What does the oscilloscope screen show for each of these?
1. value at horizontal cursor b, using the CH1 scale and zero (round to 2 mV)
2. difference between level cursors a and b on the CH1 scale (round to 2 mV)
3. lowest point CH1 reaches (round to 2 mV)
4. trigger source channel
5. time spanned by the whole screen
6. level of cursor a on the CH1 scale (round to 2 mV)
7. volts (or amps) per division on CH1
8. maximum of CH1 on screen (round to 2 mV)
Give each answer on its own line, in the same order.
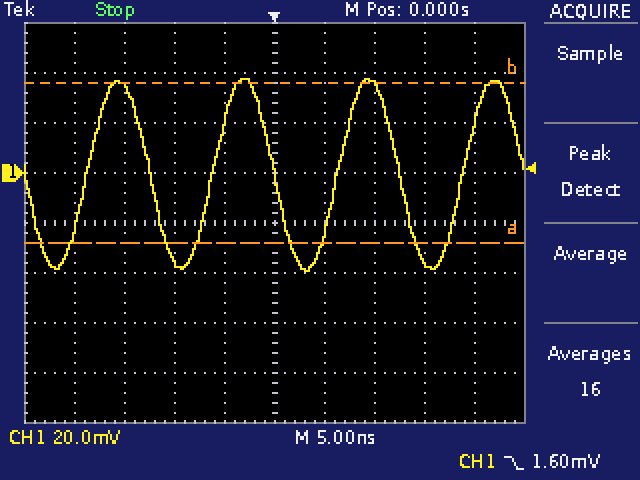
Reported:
36 mV
64 mV
-40 mV
CH1
50 ns
-28 mV
20 mV
38 mV
